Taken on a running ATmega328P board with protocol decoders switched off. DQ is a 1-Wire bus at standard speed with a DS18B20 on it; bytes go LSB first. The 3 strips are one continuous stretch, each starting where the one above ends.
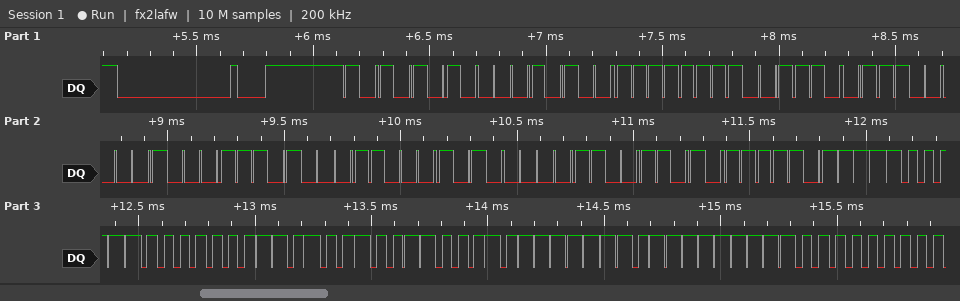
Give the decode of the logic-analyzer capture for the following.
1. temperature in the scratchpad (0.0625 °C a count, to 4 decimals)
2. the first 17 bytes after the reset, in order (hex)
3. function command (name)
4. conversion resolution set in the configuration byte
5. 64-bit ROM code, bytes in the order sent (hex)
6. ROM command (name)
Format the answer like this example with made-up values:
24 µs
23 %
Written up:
24.9375 °C
55 28 FF 9C 83 B8 18 05 B3 BE 8F 01 4B 46 7F FF 01
Read Scratchpad
12 bits
28 FF 9C 83 B8 18 05 B3
Match ROM
